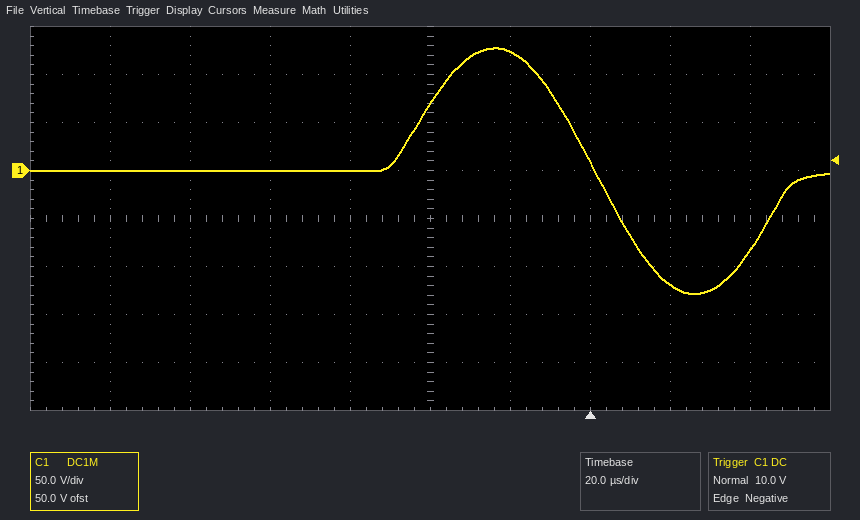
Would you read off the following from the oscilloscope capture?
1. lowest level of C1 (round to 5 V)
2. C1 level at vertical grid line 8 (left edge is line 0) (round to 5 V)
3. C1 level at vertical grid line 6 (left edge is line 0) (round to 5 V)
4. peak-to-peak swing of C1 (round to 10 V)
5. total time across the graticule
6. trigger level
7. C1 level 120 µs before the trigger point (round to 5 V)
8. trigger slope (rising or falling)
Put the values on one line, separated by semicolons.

-130 V; -120 V; 125 V; 260 V; 200 µs; 10.0 V; 0 V; falling
